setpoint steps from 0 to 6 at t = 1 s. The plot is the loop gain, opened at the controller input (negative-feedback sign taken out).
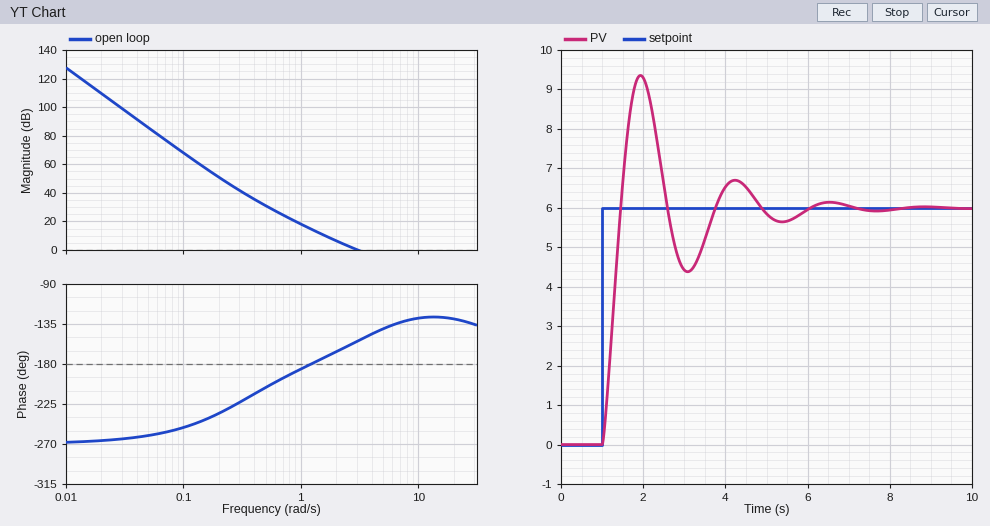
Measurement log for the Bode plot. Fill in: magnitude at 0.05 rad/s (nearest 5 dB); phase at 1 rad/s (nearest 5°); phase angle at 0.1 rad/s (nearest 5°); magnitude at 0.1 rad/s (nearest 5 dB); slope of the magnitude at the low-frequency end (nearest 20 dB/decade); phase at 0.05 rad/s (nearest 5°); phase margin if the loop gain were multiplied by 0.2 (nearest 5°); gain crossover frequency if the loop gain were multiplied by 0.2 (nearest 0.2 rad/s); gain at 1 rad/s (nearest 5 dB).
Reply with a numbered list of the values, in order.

1. 85 dB
2. -185°
3. -250°
4. 70 dB
5. -60 dB/decade
6. -260°
7. 0°
8. 1.2 rad/s
9. 20 dB
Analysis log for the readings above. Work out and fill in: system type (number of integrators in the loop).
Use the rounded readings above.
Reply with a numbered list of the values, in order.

1. 3
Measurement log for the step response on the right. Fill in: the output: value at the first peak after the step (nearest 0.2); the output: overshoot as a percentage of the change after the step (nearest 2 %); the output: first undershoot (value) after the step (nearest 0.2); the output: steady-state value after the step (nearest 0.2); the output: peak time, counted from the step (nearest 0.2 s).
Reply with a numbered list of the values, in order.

1. 9.4
2. 56 %
3. 4.4
4. 6.0
5. 1.0 s
